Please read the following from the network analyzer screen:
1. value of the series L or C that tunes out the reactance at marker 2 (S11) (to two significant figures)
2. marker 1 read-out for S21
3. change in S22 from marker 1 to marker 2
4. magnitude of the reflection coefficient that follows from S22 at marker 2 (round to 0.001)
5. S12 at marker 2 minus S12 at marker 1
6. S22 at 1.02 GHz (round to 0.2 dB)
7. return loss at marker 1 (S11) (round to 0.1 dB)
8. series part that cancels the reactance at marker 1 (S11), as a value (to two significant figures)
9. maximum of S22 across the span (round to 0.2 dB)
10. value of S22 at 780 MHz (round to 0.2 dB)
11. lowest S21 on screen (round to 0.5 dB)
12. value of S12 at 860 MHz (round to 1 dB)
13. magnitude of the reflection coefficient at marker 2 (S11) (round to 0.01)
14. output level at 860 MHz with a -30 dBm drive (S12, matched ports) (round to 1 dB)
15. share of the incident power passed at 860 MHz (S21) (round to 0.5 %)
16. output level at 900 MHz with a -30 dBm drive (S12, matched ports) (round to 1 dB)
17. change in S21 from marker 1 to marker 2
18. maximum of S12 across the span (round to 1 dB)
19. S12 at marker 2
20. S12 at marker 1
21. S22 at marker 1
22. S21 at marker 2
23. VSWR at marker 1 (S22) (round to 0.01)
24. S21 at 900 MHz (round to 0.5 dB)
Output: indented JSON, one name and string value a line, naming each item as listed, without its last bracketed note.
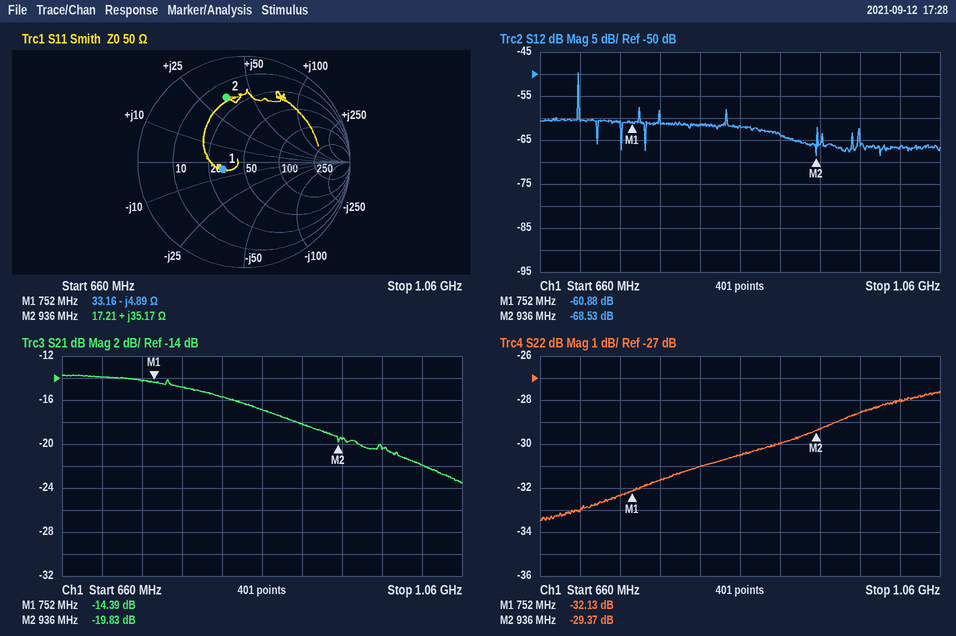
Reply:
{
  "value of the series L or C that tunes out the reactance at marker 2 (S11)": "4.8 pF",
  "marker 1 read-out for S21": "-14.39 dB",
  "change in S22 from marker 1 to marker 2": "2.76 dB",
  "magnitude of the reflection coefficient that follows from S22 at marker 2": "0.034",
  "S12 at marker 2 minus S12 at marker 1": "-7.65 dB",
  "S22 at 1.02 GHz": "-28.0 dB",
  "return loss at marker 1 (S11)": "13.5 dB",
  "series part that cancels the reactance at marker 1 (S11), as a value": "1.0 nH",
  "maximum of S22 across the span": "-27.6 dB",
  "value of S22 at 780 MHz": "-31.6 dB",
  "lowest S21 on screen": "-23.5 dB",
  "value of S12 at 860 MHz": "-62 dB",
  "magnitude of the reflection coefficient at marker 2 (S11)": "0.63",
  "output level at 860 MHz with a -30 dBm drive (S12, matched ports)": "-92 dBm",
  "share of the incident power passed at 860 MHz (S21)": "2.0 %",
  "output level at 900 MHz with a -30 dBm drive (S12, matched ports)": "-94 dBm",
  "change in S21 from marker 1 to marker 2": "-5.44 dB",
  "maximum of S12 across the span": "-50 dB",
  "S12 at marker 2": "-68.53 dB",
  "S12 at marker 1": "-60.88 dB",
  "S22 at marker 1": "-32.13 dB",
  "S21 at marker 2": "-19.83 dB",
  "VSWR at marker 1 (S22)": "1.05",
  "S21 at 900 MHz": "-18.0 dB"
}
